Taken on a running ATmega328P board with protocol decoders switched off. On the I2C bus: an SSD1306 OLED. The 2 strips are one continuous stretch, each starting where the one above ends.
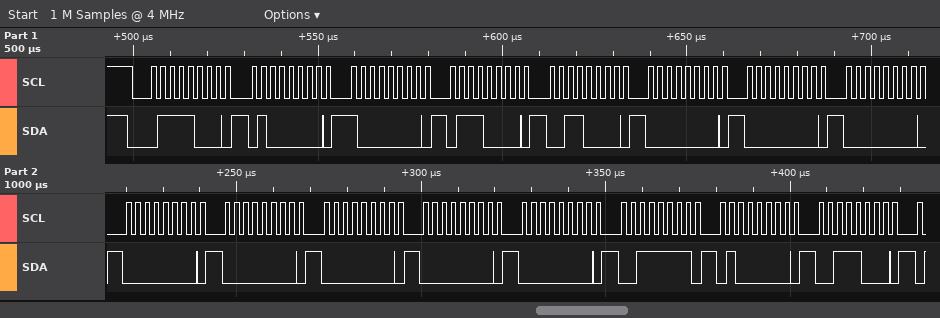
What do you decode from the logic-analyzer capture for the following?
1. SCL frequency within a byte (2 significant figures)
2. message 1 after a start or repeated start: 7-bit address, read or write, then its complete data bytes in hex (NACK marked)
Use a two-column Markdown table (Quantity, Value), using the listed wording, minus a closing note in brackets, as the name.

| Quantity | Value |
|---|---|
| SCL frequency within a byte | 400 kHz |
| message 1 after a start or repeated start: 7-bit address, read or write, then its complete data bytes in hex | 0x3C write: 40 80 70 30 00 00 00 00 00 00 00 00 3F 40 38 |
